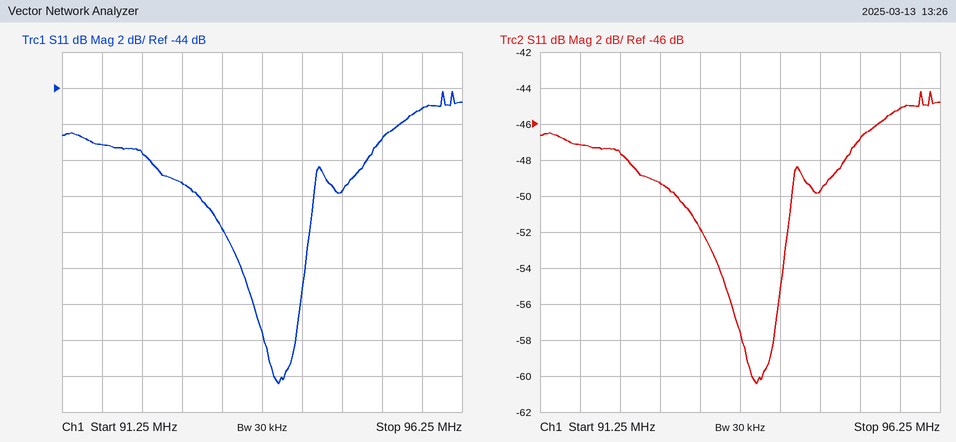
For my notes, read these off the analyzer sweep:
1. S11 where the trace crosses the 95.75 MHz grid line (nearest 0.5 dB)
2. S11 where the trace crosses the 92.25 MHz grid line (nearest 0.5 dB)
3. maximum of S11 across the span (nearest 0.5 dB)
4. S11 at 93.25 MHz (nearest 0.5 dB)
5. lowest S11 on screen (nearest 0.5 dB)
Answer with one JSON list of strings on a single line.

["-45.0 dB", "-47.5 dB", "-44.0 dB", "-52.0 dB", "-60.5 dB"]
